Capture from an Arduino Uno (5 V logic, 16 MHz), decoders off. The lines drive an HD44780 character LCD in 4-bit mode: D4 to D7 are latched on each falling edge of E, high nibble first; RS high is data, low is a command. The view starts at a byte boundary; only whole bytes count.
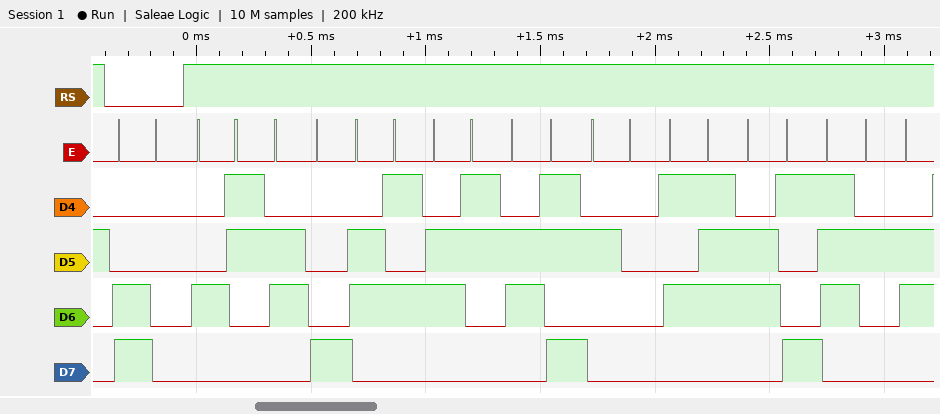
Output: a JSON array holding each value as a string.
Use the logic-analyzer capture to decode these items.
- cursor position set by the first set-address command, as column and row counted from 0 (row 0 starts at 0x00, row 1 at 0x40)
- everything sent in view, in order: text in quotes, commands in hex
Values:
["column 0, row 1", "0xC0 \"Check Wir\""]
